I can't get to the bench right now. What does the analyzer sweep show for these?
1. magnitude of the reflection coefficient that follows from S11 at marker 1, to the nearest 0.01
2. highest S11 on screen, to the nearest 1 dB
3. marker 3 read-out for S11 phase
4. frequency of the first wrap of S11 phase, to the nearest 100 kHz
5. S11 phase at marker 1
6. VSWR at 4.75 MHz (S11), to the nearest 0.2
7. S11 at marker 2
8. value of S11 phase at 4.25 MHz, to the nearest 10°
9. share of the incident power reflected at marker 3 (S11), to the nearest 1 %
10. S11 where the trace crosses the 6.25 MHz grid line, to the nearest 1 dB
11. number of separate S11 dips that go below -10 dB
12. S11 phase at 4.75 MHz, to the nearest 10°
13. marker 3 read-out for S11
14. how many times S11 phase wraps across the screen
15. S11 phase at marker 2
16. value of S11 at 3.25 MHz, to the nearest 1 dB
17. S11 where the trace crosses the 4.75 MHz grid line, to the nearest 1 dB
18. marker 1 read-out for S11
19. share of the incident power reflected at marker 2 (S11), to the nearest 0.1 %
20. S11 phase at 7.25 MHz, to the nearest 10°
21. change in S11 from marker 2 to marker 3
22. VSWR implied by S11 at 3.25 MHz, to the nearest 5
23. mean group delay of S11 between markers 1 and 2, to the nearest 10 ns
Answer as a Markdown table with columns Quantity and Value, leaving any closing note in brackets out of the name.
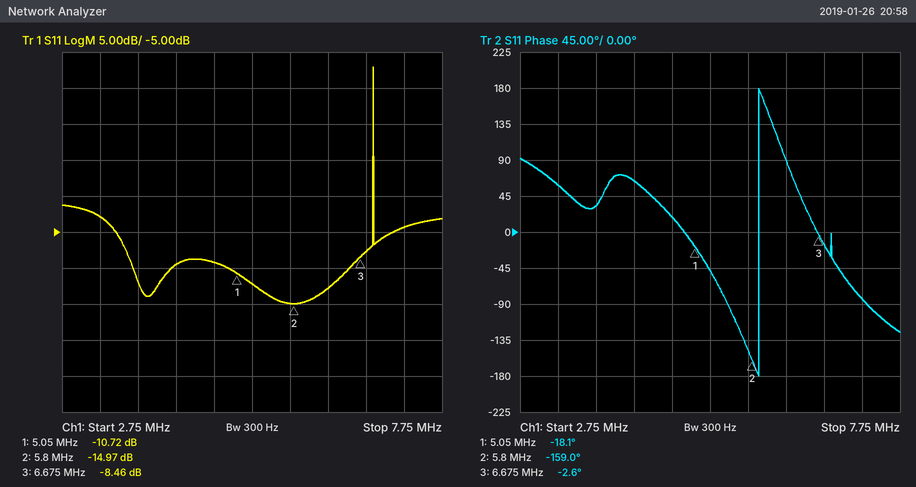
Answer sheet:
| Quantity | Value |
|---|---|
| magnitude of the reflection coefficient that follows from S11 at marker 1, to the nearest 0.01 | 0.29 |
| highest S11 on screen, to the nearest 1 dB | 18 dB |
| marker 3 read-out for S11 phase | -2.6° |
| frequency of the first wrap of S11 phase, to the nearest 100 kHz | 5.9 MHz |
| S11 phase at marker 1 | -18.1° |
| VSWR at 4.75 MHz (S11), to the nearest 0.2 | 2.0 |
| S11 at marker 2 | -14.97 dB |
| value of S11 phase at 4.25 MHz, to the nearest 10° | 60° |
| share of the incident power reflected at marker 3 (S11), to the nearest 1 % | 14 % |
| S11 where the trace crosses the 6.25 MHz grid line, to the nearest 1 dB | -13 dB |
| number of separate S11 dips that go below -10 dB | 2 |
| S11 phase at 4.75 MHz, to the nearest 10° | 20° |
| marker 3 read-out for S11 | -8.46 dB |
| how many times S11 phase wraps across the screen | 1 |
| S11 phase at marker 2 | -159.0° |
| value of S11 at 3.25 MHz, to the nearest 1 dB | -3 dB |
| S11 where the trace crosses the 4.75 MHz grid line, to the nearest 1 dB | -9 dB |
| marker 1 read-out for S11 | -10.72 dB |
| share of the incident power reflected at marker 2 (S11), to the nearest 0.1 % | 3.2 % |
| S11 phase at 7.25 MHz, to the nearest 10° | -80° |
| change in S11 from marker 2 to marker 3 | 6.51 dB |
| VSWR implied by S11 at 3.25 MHz, to the nearest 5 | 5 |
| mean group delay of S11 between markers 1 and 2, to the nearest 10 ns | 520 ns |
